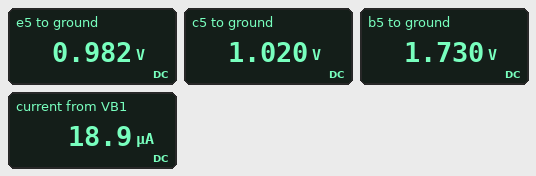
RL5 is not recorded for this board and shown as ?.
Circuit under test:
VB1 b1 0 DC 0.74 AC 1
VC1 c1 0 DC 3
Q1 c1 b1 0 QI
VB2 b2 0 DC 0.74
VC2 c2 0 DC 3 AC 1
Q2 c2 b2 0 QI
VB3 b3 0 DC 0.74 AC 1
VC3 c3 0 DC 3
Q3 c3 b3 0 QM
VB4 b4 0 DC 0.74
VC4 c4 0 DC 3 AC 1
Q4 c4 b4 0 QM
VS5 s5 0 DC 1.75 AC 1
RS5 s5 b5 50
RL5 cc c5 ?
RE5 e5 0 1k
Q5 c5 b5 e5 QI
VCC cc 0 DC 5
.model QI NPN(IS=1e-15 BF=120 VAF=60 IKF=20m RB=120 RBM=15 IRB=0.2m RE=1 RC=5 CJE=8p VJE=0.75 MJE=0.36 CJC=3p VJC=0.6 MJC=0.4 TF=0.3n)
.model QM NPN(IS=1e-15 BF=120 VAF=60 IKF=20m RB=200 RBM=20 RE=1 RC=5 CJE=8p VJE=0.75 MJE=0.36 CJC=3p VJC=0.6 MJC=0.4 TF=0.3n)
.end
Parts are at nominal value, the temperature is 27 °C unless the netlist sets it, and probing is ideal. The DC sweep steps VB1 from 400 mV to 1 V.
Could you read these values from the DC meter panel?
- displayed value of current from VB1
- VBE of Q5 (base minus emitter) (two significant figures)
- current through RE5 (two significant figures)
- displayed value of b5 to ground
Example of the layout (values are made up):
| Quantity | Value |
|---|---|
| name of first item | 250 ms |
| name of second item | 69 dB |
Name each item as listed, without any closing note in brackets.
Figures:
| Quantity | Value |
|---|---|
| displayed value of current from VB1 | 18.9 µA |
| VBE of Q5 (base minus emitter) | 750 mV |
| current through RE5 | 980 µA |
| displayed value of b5 to ground | 1.730 V |
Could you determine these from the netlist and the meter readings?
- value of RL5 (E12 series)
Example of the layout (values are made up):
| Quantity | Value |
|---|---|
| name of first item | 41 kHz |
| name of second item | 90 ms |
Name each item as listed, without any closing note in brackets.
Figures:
| Quantity | Value |
|---|---|
| value of RL5 | 6.8 kΩ |
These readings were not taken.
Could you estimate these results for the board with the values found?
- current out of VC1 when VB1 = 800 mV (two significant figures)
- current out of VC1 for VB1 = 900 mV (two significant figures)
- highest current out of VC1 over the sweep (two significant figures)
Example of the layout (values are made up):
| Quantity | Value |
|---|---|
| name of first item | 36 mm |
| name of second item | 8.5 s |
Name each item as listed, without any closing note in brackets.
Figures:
| Quantity | Value |
|---|---|
| current out of VC1 when VB1 = 800 mV | 9.5 mA |
| current out of VC1 for VB1 = 900 mV | 34 mA |
| highest current out of VC1 over the sweep | 63 mA |
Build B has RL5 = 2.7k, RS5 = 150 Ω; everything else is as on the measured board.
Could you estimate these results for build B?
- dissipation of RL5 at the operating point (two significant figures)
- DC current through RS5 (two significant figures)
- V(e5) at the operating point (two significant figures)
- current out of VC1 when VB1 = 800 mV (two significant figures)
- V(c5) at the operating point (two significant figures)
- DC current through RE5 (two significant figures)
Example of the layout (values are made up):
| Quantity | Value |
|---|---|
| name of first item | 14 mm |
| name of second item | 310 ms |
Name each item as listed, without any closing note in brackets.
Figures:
| Quantity | Value |
|---|---|
| dissipation of RL5 at the operating point | 2.8 mW |
| DC current through RS5 | 8.9 µA |
| V(e5) at the operating point | 1.0 V |
| current out of VC1 when VB1 = 800 mV | 9.5 mA |
| V(c5) at the operating point | 2.2 V |
| DC current through RE5 | 1.0 mA |
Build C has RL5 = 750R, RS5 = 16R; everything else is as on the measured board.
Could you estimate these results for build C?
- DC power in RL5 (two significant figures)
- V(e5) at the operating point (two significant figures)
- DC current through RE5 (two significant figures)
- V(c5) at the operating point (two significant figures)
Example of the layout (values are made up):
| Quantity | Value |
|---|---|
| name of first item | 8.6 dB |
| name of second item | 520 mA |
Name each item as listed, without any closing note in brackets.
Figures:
| Quantity | Value |
|---|---|
| DC power in RL5 | 790 µW |
| V(e5) at the operating point | 1.0 V |
| DC current through RE5 | 1.0 mA |
| V(c5) at the operating point | 4.2 V |
